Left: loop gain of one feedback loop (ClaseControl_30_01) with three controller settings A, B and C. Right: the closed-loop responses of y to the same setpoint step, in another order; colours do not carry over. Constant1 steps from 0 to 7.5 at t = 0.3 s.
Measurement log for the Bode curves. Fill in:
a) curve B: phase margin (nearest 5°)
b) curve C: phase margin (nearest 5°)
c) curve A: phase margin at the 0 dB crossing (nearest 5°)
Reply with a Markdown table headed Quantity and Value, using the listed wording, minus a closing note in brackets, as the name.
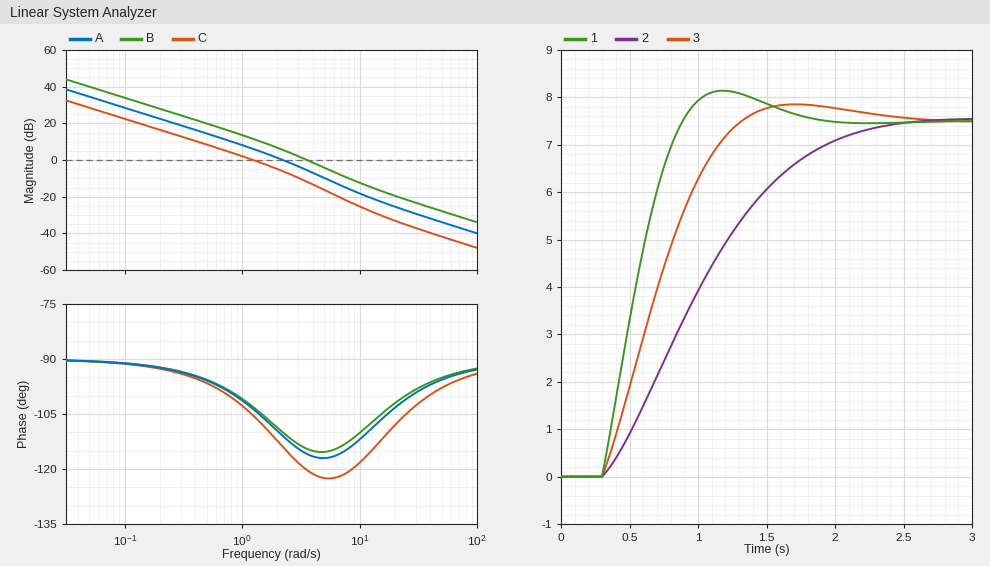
| Quantity | Value |
|---|---|
| curve B: phase margin | 65° |
| curve C: phase margin | 75° |
| curve A: phase margin at the 0 dB crossing | 70° |
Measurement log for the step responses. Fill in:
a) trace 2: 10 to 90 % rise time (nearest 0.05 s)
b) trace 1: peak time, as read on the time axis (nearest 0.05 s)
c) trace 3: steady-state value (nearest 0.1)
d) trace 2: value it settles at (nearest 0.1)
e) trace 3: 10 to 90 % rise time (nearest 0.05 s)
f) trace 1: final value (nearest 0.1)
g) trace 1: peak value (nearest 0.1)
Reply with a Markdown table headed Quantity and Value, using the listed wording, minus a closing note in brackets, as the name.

| Quantity | Value |
|---|---|
| trace 2: 10 to 90 % rise time | 1.30 s |
| trace 1: peak time, as read on the time axis | 1.20 s |
| trace 3: steady-state value | 7.5 |
| trace 2: value it settles at | 7.5 |
| trace 3: 10 to 90 % rise time | 0.70 s |
| trace 1: final value | 7.5 |
| trace 1: peak value | 8.1 |
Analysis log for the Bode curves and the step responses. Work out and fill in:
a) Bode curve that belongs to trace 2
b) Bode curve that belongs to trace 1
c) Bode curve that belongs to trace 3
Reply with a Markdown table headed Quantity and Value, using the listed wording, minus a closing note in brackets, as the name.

| Quantity | Value |
|---|---|
| Bode curve that belongs to trace 2 | C |
| Bode curve that belongs to trace 1 | B |
| Bode curve that belongs to trace 3 | A |
